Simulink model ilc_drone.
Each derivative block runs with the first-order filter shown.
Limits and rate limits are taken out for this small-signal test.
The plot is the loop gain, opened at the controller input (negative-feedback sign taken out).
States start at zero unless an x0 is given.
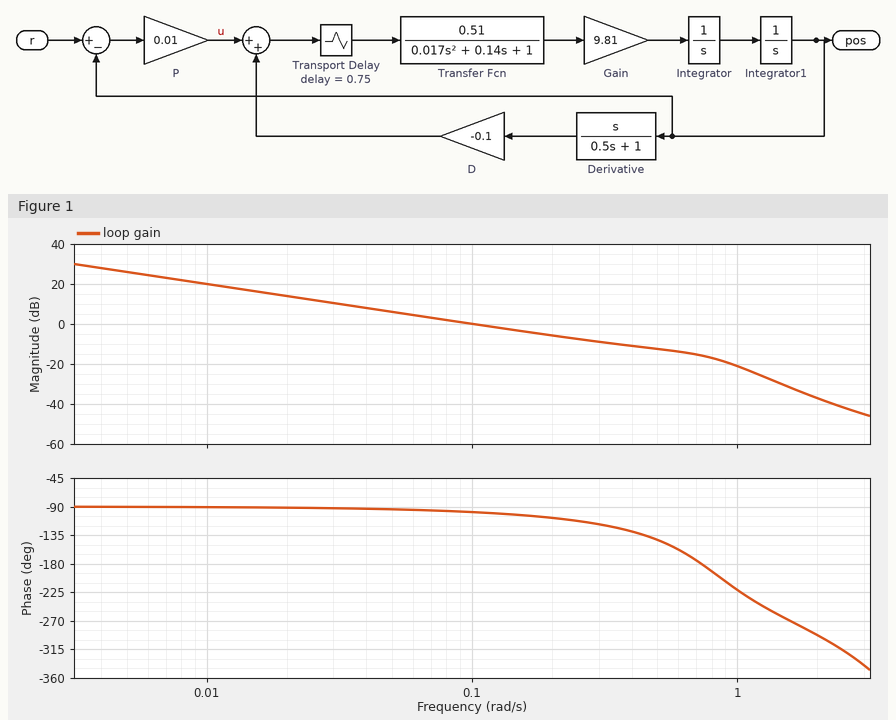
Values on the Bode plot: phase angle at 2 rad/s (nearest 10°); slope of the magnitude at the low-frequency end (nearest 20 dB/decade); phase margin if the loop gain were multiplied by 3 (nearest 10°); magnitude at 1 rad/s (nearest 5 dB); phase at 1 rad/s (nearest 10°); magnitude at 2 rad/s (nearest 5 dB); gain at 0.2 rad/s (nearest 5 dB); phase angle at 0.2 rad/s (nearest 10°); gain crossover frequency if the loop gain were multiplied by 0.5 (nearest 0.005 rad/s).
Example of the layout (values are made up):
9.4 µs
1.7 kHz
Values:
-290°
-20 dB/decade
60°
-20 dB
-220°
-35 dB
-5 dB
-110°
0.050 rad/s
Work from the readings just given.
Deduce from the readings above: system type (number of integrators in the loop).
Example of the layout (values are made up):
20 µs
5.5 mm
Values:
1
